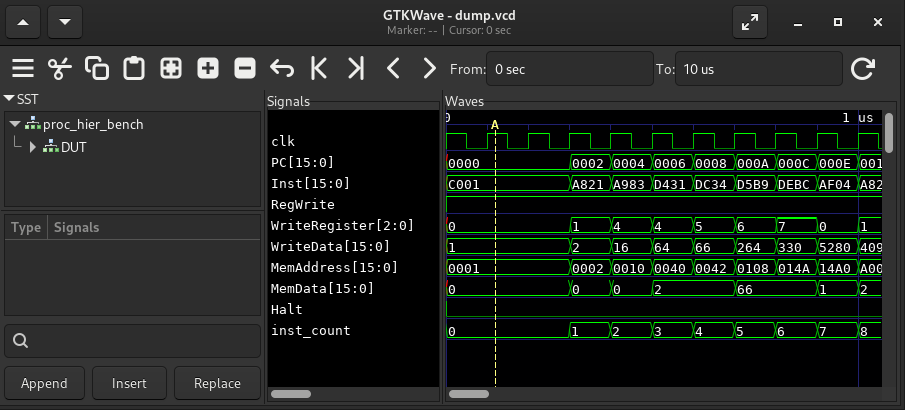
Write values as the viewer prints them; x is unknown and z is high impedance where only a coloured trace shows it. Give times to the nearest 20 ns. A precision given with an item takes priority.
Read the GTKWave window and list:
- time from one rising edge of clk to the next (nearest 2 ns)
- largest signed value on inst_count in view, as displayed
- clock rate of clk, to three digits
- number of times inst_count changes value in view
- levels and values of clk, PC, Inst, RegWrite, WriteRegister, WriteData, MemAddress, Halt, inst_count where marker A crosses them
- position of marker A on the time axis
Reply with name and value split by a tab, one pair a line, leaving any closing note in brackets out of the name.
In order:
time from one rising edge of clk to the next	100 ns
largest signed value on inst_count in view, as displayed	8
clock rate of clk, to three digits	10.0 MHz
number of times inst_count changes value in view	8
levels and values of clk, PC, Inst, RegWrite, WriteRegister, WriteData, MemAddress, Halt, inst_count where marker A crosses them	clk=1, PC=0000, Inst=C001, RegWrite=1, WriteRegister=0, WriteData=1, MemAddress=0001, Halt=0, inst_count=0
position of marker A on the time axis	120 ns
